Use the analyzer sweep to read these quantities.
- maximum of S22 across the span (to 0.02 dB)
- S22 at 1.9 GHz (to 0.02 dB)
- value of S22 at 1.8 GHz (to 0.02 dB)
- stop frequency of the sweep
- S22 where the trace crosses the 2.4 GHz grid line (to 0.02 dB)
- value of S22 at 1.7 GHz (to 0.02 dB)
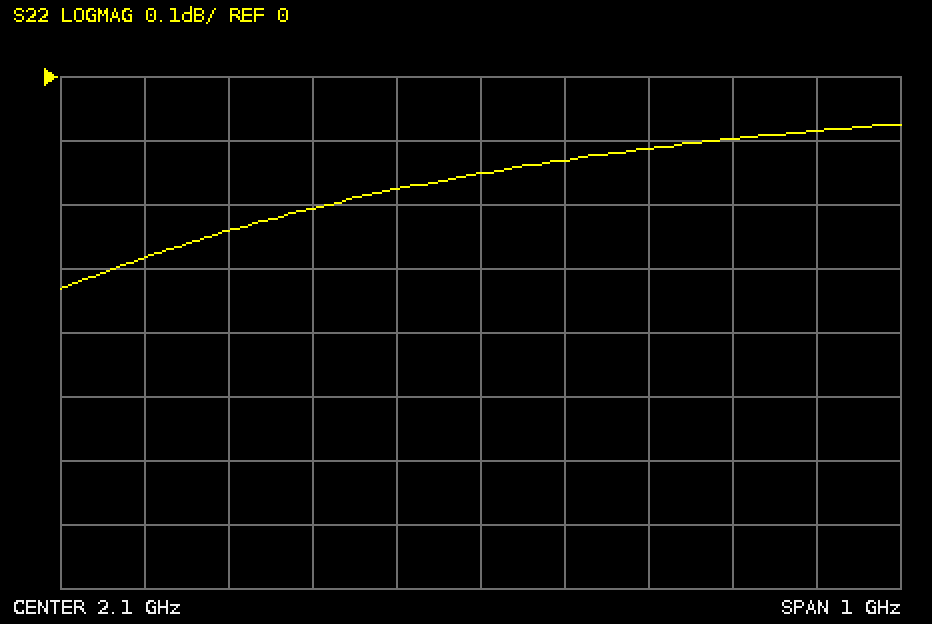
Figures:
-0.08 dB
-0.20 dB
-0.24 dB
2.6 GHz
-0.10 dB
-0.28 dB
